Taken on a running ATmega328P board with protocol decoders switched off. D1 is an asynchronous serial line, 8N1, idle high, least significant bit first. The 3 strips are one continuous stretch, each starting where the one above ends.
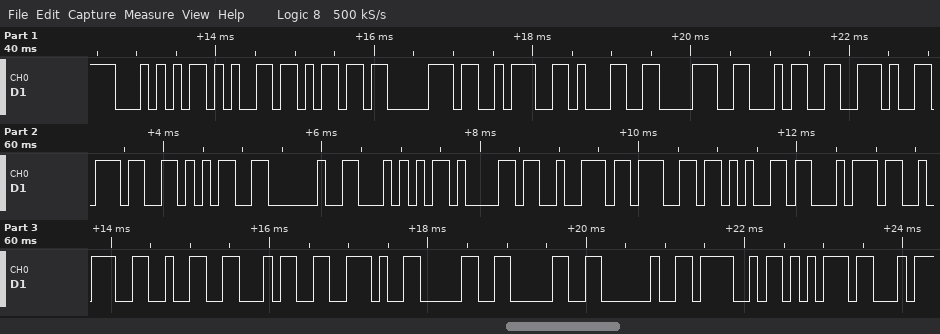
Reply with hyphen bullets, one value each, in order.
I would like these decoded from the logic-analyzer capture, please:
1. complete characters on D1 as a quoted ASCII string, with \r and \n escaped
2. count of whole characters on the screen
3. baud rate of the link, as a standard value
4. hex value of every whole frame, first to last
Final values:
- "Temp:184.75 Target:24.00 Ou"
- 27
- 9600 baud
- 54 65 6D 70 3A 31 38 34 2E 37 35 20 54 61 72 67 65 74 3A 32 34 2E 30 30 20 4F 75
